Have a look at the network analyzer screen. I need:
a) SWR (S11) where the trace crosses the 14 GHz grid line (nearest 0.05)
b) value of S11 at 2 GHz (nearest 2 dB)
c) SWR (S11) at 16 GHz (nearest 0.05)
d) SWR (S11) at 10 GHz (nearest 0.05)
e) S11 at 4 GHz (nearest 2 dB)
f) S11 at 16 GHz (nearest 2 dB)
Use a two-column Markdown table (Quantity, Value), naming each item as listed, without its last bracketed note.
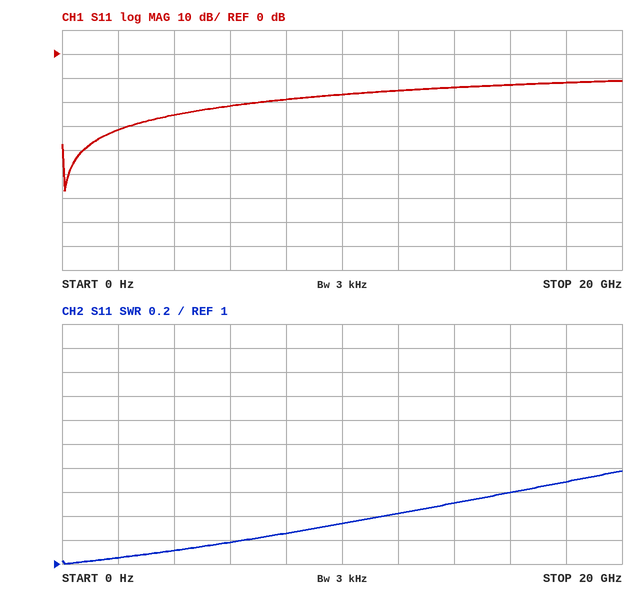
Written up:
| Quantity | Value |
|---|---|
| SWR (S11) where the trace crosses the 14 GHz grid line | 1.50 |
| value of S11 at 2 GHz | -32 dB |
| SWR (S11) at 16 GHz | 1.60 |
| SWR (S11) at 10 GHz | 1.35 |
| S11 at 4 GHz | -26 dB |
| S11 at 16 GHz | -12 dB |
